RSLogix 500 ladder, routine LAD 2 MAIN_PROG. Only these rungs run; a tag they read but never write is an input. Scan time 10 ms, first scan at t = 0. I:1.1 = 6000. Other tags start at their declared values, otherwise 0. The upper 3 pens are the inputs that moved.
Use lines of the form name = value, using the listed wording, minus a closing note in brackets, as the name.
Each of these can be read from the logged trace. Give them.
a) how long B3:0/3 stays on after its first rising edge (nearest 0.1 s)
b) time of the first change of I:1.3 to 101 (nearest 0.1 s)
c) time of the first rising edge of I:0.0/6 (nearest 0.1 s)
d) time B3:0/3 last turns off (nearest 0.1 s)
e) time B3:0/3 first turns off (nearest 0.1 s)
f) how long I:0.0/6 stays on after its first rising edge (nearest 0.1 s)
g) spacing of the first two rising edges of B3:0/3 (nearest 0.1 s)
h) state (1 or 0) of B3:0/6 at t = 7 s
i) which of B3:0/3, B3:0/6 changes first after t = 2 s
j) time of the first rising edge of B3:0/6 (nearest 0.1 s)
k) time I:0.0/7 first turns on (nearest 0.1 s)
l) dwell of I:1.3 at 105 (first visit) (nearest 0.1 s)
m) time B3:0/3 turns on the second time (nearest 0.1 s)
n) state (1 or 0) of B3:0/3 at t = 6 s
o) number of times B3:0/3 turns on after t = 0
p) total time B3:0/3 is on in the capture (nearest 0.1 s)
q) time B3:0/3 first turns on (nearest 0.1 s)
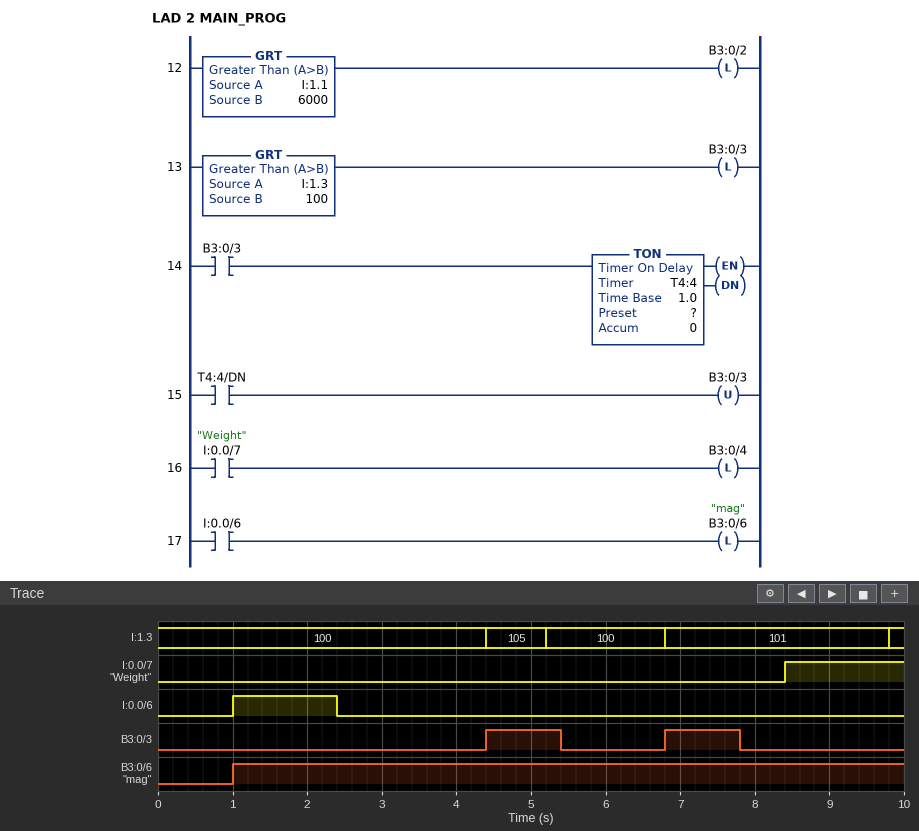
how long B3:0/3 stays on after its first rising edge = 1.0 s
time of the first change of I:1.3 to 101 = 6.8 s
time of the first rising edge of I:0.0/6 = 1.0 s
time B3:0/3 last turns off = 7.8 s
time B3:0/3 first turns off = 5.4 s
how long I:0.0/6 stays on after its first rising edge = 1.4 s
spacing of the first two rising edges of B3:0/3 = 2.4 s
state (1 or 0) of B3:0/6 at t = 7 s = 1
which of B3:0/3, B3:0/6 changes first after t = 2 s = B3:0/3
time of the first rising edge of B3:0/6 = 1.0 s
time I:0.0/7 first turns on = 8.4 s
dwell of I:1.3 at 105 (first visit) = 0.8 s
time B3:0/3 turns on the second time = 6.8 s
state (1 or 0) of B3:0/3 at t = 6 s = 0
number of times B3:0/3 turns on after t = 0 = 2
total time B3:0/3 is on in the capture = 2.0 s
time B3:0/3 first turns on = 4.4 s
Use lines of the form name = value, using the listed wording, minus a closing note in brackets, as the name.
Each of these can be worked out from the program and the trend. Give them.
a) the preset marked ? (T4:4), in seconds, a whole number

the preset marked ? (T4:4), in seconds, a whole number = 1 s
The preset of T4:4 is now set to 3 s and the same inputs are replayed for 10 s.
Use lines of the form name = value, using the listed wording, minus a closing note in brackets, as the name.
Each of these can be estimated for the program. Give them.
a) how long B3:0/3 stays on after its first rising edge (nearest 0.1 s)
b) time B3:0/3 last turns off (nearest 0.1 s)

how long B3:0/3 stays on after its first rising edge = 3.0 s
time B3:0/3 last turns off = 7.4 s
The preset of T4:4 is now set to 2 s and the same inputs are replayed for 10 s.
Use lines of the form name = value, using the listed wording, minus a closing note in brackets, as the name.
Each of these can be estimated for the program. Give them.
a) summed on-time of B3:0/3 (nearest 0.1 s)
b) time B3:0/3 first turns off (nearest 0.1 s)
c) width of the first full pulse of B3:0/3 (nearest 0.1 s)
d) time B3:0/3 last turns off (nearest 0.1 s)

summed on-time of B3:0/3 = 4.0 s
time B3:0/3 first turns off = 6.4 s
width of the first full pulse of B3:0/3 = 2.0 s
time B3:0/3 last turns off = 8.8 s
